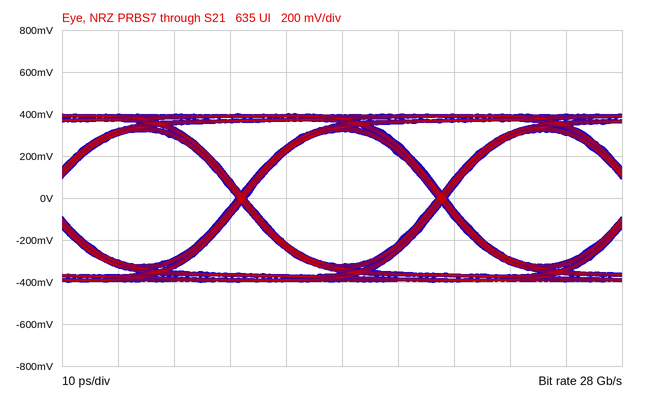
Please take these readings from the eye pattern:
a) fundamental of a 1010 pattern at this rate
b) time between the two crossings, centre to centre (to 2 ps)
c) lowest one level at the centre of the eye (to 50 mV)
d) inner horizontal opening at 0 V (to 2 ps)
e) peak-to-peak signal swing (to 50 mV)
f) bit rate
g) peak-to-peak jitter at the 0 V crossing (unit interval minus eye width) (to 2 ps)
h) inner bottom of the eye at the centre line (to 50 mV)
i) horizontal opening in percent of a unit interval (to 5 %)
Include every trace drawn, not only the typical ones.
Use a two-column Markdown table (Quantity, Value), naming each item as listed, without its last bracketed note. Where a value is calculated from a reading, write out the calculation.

| Quantity | Value |
|---|---|
| fundamental of a 1010 pattern at this rate | 14 GHz |
| time between the two crossings, centre to centre | 36 ps |
| lowest one level at the centre of the eye | 300 mV |
| inner horizontal opening at 0 V | 34 ps |
| peak-to-peak signal swing | 800 mV |
| bit rate | 28 Gb/s |
| peak-to-peak jitter at the 0 V crossing (unit interval minus eye width) | 2 ps |
| inner bottom of the eye at the centre line | -300 mV |
| horizontal opening in percent of a unit interval | 34 ps / 36 ps ≈ 94.4 %, so 95 % to the nearest 5 % |
